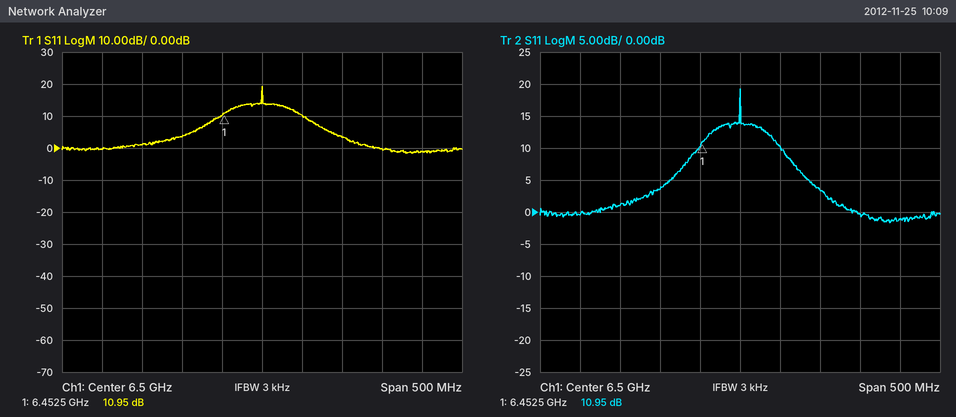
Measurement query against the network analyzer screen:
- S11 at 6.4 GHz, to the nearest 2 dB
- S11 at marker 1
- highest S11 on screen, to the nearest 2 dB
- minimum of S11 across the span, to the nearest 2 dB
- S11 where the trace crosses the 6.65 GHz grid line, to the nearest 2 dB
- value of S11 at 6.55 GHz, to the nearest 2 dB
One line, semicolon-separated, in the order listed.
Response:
4 dB; 10.95 dB; 20 dB; -2 dB; 0 dB; 10 dB
